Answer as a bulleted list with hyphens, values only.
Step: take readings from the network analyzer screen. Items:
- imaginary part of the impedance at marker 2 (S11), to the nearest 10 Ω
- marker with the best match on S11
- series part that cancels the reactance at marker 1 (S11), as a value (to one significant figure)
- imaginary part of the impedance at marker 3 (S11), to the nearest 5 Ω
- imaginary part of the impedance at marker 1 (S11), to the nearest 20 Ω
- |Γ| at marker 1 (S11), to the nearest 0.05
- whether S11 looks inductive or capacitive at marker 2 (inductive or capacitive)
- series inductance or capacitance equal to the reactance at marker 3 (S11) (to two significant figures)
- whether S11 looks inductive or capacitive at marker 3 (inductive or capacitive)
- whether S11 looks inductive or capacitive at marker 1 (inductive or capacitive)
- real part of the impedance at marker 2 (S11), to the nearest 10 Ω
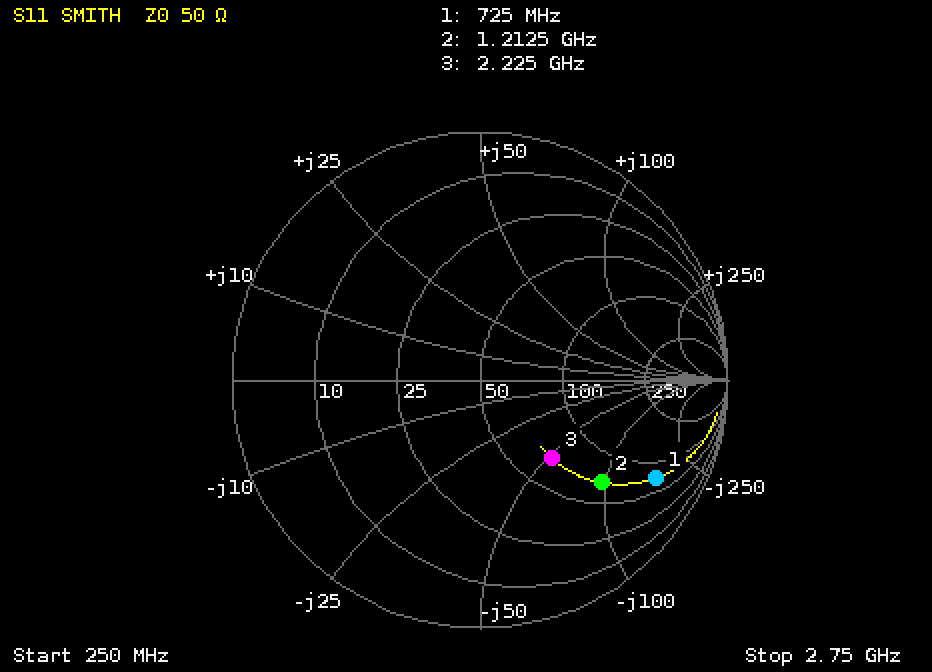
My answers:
- -100 Ω
- marker 3
- 40 nH
- -50 Ω
- -160 Ω
- 0.80
- capacitive
- 1.4 pF
- capacitive
- capacitive
- 70 Ω
